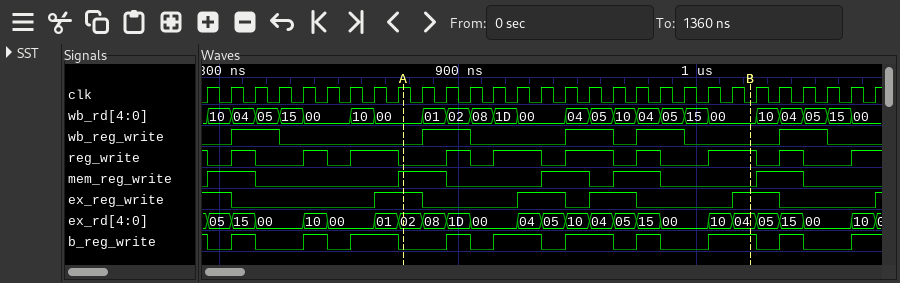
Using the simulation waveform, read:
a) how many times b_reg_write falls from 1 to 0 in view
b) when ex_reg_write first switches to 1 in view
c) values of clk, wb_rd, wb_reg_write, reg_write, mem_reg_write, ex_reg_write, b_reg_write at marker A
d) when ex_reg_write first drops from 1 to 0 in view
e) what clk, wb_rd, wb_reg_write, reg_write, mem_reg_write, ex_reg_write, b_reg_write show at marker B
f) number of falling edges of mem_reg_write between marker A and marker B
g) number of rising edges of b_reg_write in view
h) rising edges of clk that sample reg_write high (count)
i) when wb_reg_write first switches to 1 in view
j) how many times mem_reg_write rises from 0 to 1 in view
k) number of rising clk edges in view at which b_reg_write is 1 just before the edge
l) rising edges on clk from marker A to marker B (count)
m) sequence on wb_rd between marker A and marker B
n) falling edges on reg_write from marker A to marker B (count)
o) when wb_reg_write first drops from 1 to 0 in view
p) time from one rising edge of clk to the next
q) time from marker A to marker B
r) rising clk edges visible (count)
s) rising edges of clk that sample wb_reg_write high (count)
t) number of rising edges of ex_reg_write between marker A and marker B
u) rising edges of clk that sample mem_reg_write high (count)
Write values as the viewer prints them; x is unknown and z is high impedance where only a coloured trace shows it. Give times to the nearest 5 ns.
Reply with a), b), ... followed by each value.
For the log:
a) 10
b) 865 ns
c) clk=1, wb_rd=00, wb_reg_write=0, reg_write=0, mem_reg_write=1, ex_reg_write=1, b_reg_write=0
d) 805 ns
e) clk=0, wb_rd=00, wb_reg_write=0, reg_write=1, mem_reg_write=0, ex_reg_write=1, b_reg_write=1
f) 3
g) 10
h) 15
i) 805 ns
j) 5
k) 15
l) 14
m) 00, 01, 02, 08, 1D, 00, 04, 05, 10, 04, 05, 15, 00
n) 4
o) 825 ns
p) 10 ns
q) 145 ns
r) 29
s) 10
t) 3
u) 10
